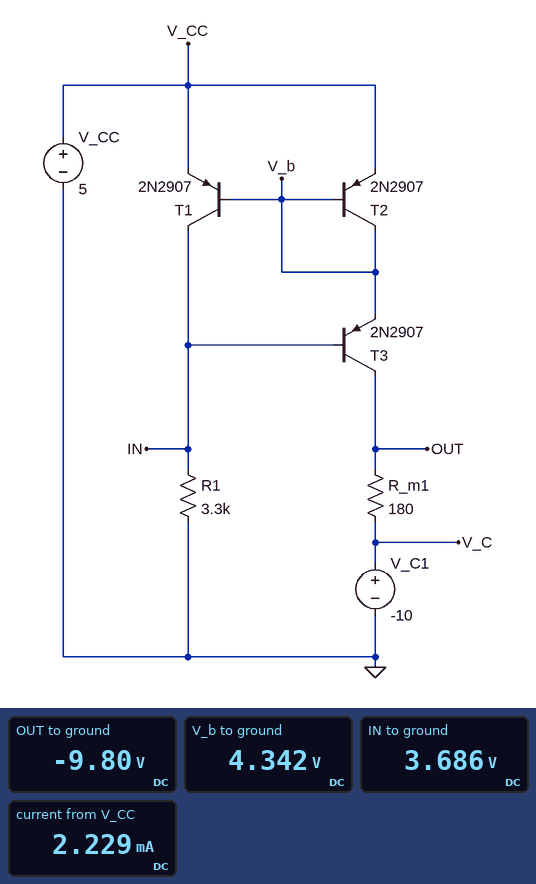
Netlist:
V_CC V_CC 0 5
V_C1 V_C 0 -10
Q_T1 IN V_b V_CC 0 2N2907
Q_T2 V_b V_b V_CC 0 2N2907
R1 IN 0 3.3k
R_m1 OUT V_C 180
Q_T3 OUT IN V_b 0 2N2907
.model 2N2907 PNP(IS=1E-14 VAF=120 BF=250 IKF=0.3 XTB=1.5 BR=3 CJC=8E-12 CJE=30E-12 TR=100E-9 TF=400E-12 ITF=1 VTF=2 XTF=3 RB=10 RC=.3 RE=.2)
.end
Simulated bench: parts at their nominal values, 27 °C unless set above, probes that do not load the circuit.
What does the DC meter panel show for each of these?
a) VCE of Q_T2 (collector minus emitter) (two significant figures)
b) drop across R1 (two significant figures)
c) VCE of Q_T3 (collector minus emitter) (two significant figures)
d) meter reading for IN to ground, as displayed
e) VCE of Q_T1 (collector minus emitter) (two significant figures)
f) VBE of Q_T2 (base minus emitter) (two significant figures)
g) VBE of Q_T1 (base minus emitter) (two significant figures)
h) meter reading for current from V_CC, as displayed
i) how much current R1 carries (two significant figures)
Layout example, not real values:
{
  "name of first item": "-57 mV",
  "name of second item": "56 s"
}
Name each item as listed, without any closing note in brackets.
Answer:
{
  "VCE of Q_T2 (collector minus emitter)": "-660 mV",
  "drop across R1": "3.7 V",
  "VCE of Q_T3 (collector minus emitter)": "-14 V",
  "meter reading for IN to ground, as displayed": "3.686 V",
  "VCE of Q_T1 (collector minus emitter)": "-1.3 V",
  "VBE of Q_T2 (base minus emitter)": "-660 mV",
  "VBE of Q_T1 (base minus emitter)": "-660 mV",
  "meter reading for current from V_CC, as displayed": "2.229 mA",
  "how much current R1 carries": "1.1 mA"
}
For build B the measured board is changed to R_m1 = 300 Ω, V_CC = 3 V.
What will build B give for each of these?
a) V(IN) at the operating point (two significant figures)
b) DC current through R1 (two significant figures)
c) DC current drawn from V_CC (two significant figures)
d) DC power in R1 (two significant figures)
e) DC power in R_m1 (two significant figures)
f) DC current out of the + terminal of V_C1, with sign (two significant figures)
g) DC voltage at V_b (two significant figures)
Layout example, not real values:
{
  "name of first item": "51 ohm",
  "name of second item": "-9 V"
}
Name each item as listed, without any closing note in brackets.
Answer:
{
  "V(IN) at the operating point": "1.7 V",
  "DC current through R1": "520 µA",
  "DC current drawn from V_CC": "1.0 mA",
  "DC power in R1": "900 µW",
  "DC power in R_m1": "81 µW",
  "DC current out of the + terminal of V_C1, with sign": "-520 µA",
  "DC voltage at V_b": "2.4 V"
}
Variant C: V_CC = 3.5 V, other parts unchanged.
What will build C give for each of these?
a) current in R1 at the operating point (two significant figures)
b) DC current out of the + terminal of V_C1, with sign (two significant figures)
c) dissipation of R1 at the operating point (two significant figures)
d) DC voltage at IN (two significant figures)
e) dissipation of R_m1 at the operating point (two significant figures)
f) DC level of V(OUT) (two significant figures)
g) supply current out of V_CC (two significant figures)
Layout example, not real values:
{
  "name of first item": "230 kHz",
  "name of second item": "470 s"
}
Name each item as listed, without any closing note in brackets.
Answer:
{
  "current in R1 at the operating point": "670 µA",
  "DC current out of the + terminal of V_C1, with sign": "-670 µA",
  "dissipation of R1 at the operating point": "1.5 mW",
  "DC voltage at IN": "2.2 V",
  "dissipation of R_m1 at the operating point": "80 µW",
  "DC level of V(OUT)": "-9.9 V",
  "supply current out of V_CC": "1.3 mA"
}
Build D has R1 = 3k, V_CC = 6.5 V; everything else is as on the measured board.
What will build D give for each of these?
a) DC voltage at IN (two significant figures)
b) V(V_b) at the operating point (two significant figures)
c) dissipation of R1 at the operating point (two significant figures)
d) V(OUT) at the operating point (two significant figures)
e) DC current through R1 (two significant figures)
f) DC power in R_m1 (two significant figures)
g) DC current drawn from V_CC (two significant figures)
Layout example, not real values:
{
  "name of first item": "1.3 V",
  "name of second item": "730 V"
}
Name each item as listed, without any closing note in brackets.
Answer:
{
  "DC voltage at IN": "5.2 V",
  "V(V_b) at the operating point": "5.8 V",
  "dissipation of R1 at the operating point": "8.9 mW",
  "V(OUT) at the operating point": "-9.7 V",
  "DC current through R1": "1.7 mA",
  "DC power in R_m1": "530 µW",
  "DC current drawn from V_CC": "3.4 mA"
}
